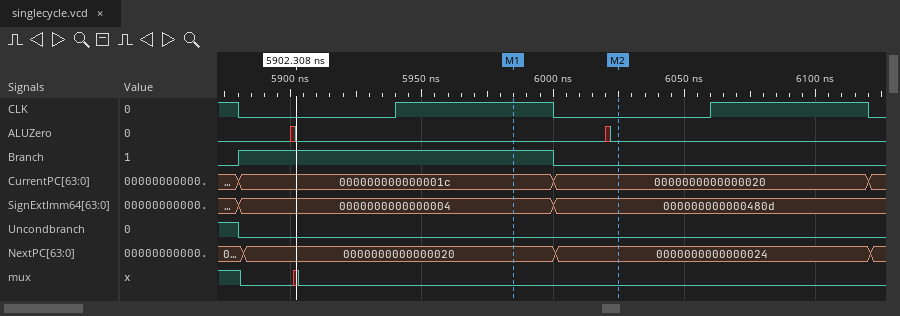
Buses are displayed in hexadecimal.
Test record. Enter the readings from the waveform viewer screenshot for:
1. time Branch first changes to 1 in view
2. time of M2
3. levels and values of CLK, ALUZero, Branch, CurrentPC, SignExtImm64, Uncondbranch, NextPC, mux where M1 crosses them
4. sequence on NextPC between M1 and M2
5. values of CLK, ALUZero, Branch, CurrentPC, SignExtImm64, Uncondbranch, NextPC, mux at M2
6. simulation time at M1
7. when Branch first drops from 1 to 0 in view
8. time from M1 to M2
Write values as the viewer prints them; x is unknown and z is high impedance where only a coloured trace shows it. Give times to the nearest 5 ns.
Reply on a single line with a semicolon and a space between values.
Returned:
5880 ns; 6025 ns; CLK=1, ALUZero=0, Branch=1, CurrentPC=000000000000001c, SignExtImm64=0000000000000004, Uncondbranch=0, NextPC=0000000000000020, mux=0; 0000000000000020, 0000000000000024; CLK=0, ALUZero=0, Branch=0, CurrentPC=0000000000000020, SignExtImm64=000000000000480d, Uncondbranch=0, NextPC=0000000000000024, mux=0; 5985 ns; 6000 ns; 40 ns
